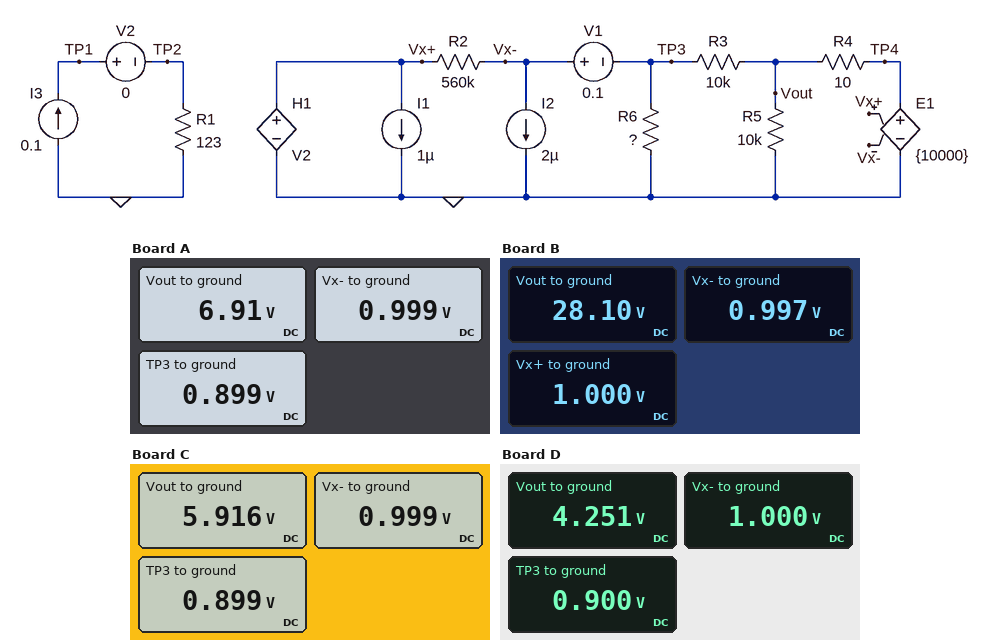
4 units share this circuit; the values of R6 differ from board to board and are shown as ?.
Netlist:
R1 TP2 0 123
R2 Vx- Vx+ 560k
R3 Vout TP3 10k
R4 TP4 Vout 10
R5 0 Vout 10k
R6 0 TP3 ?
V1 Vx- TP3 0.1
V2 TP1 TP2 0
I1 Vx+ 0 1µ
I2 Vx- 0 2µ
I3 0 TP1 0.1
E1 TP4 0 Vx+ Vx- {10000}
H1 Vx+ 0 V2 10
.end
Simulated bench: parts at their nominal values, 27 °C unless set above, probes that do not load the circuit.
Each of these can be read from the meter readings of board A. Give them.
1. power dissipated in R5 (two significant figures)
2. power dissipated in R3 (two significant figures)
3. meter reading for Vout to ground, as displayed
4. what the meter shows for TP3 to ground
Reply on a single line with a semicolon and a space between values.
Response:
4.8 mW; 3.6 mW; 6.91 V; 0.899 V
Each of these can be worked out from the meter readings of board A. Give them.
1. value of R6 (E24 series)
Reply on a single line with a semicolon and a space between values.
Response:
1.5 kΩ
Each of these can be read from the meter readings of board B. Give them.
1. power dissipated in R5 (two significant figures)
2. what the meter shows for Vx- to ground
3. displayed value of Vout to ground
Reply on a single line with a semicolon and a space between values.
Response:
79 mW; 0.997 V; 28.10 V
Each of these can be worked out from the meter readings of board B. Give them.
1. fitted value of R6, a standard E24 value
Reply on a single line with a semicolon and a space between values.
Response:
330 Ω
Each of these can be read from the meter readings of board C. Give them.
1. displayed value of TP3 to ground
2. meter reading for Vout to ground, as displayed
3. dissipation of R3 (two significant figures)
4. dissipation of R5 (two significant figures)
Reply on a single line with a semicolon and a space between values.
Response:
0.899 V; 5.916 V; 2.5 mW; 3.5 mW
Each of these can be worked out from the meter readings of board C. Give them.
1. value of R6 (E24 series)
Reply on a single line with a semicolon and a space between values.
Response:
1.8 kΩ
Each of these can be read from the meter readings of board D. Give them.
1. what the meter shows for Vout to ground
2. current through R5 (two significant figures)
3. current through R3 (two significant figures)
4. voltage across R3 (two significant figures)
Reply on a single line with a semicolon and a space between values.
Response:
4.251 V; 430 µA; 340 µA; 3.4 V
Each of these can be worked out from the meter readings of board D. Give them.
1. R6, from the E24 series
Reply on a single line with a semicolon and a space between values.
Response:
2.7 kΩ
